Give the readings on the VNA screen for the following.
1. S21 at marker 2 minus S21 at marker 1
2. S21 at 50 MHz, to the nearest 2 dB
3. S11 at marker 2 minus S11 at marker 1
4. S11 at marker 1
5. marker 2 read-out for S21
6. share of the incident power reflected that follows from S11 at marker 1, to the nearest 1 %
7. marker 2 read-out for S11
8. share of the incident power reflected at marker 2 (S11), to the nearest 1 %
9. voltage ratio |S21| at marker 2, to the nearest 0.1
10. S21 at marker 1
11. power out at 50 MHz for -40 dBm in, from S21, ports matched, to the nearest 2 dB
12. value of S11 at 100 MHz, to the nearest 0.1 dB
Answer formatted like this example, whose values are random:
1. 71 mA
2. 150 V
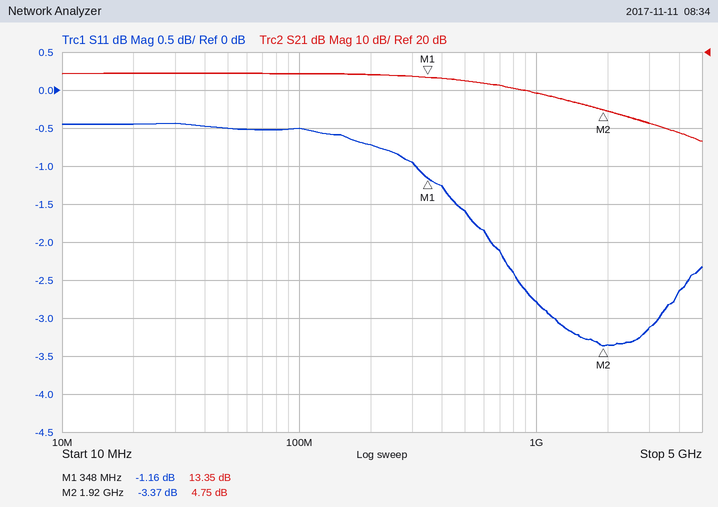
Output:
1. -8.60 dB
2. 14 dB
3. -2.21 dB
4. -1.16 dB
5. 4.75 dB
6. 77 %
7. -3.37 dB
8. 46 %
9. 1.7
10. 13.35 dB
11. -26 dBm
12. -0.5 dB
